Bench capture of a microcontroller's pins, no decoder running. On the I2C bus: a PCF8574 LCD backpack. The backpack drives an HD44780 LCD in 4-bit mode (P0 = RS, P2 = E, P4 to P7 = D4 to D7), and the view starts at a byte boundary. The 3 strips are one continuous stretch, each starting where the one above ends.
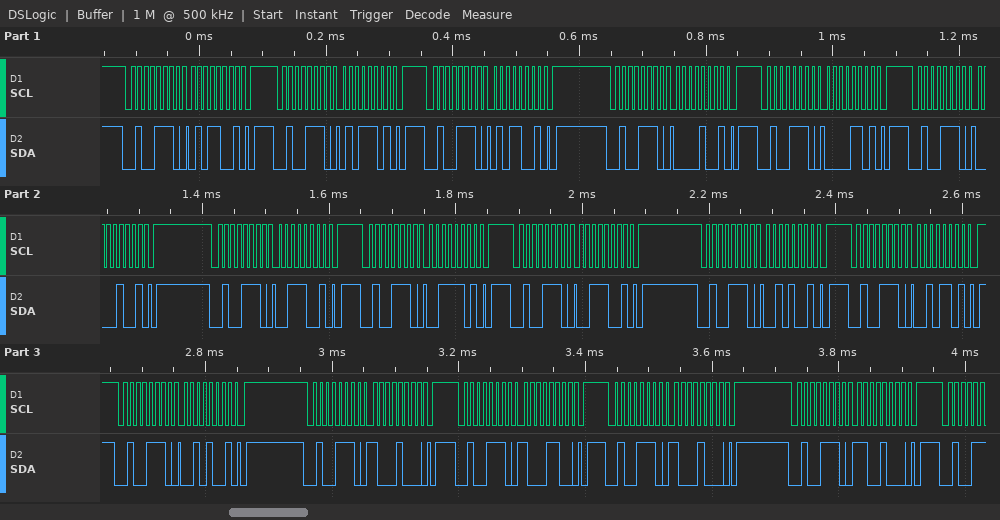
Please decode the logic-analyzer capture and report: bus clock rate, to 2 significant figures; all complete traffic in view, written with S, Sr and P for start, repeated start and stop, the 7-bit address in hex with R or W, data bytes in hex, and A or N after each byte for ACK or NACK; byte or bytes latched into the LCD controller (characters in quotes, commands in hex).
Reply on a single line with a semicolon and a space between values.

100 kHz; S 27W A 59 A P S 27W A 5D A P S 27W A 59 A P S 27W A 09 A P S 27W A 0D A P S 27W A 09 A P S 27W A 39 A P S 27W A 3D A P S 27W A 39 A P S 27W A 29 A P S 27W A 2D A P S 27W A 29 A P S 27W A 88 A P S 27W A 8C A P S 27W A 88 A P S 27W A C8 A P; 'P' '2'
